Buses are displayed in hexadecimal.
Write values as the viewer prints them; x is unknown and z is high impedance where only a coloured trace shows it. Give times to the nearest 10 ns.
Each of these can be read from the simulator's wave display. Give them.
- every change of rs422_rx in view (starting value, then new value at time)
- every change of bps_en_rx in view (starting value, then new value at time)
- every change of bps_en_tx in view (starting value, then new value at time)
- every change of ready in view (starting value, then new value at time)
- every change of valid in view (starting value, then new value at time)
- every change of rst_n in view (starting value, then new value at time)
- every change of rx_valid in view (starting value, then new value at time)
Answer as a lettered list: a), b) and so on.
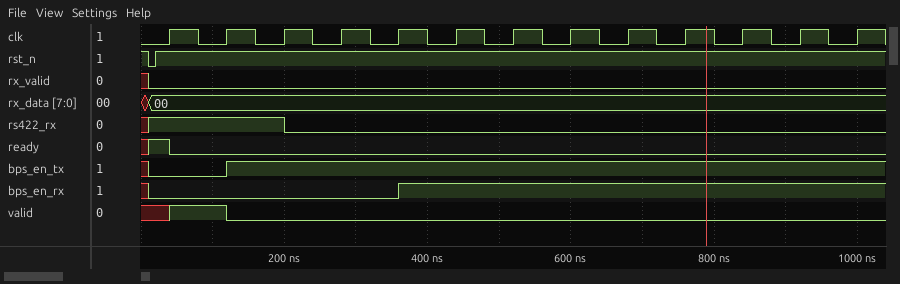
a) x, 1 at 10 ns, 0 at 200 ns
b) x, 0 at 10 ns, 1 at 360 ns
c) x, 0 at 10 ns, 1 at 120 ns
d) x, 1 at 10 ns, 0 at 40 ns
e) x, 1 at 40 ns, 0 at 120 ns
f) 1, 0 at 10 ns, 1 at 20 ns
g) x, 0 at 10 ns
